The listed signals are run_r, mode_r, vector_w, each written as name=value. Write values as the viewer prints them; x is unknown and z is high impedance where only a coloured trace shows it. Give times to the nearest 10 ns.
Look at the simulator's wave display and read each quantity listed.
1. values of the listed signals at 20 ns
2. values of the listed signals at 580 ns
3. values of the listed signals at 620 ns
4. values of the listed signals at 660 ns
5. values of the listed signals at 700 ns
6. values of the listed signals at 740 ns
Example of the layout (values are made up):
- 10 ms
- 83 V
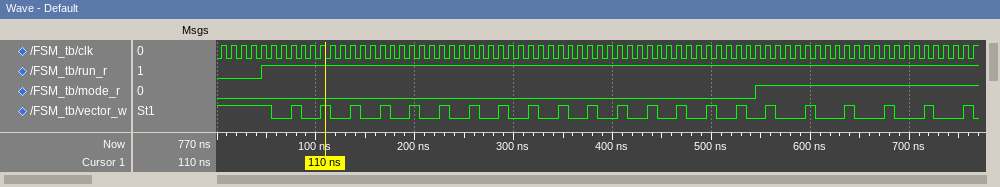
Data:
- run_r=0, mode_r=0, vector_w=1
- run_r=1, mode_r=1, vector_w=0
- run_r=1, mode_r=1, vector_w=0
- run_r=1, mode_r=1, vector_w=0
- run_r=1, mode_r=1, vector_w=0
- run_r=1, mode_r=1, vector_w=0
